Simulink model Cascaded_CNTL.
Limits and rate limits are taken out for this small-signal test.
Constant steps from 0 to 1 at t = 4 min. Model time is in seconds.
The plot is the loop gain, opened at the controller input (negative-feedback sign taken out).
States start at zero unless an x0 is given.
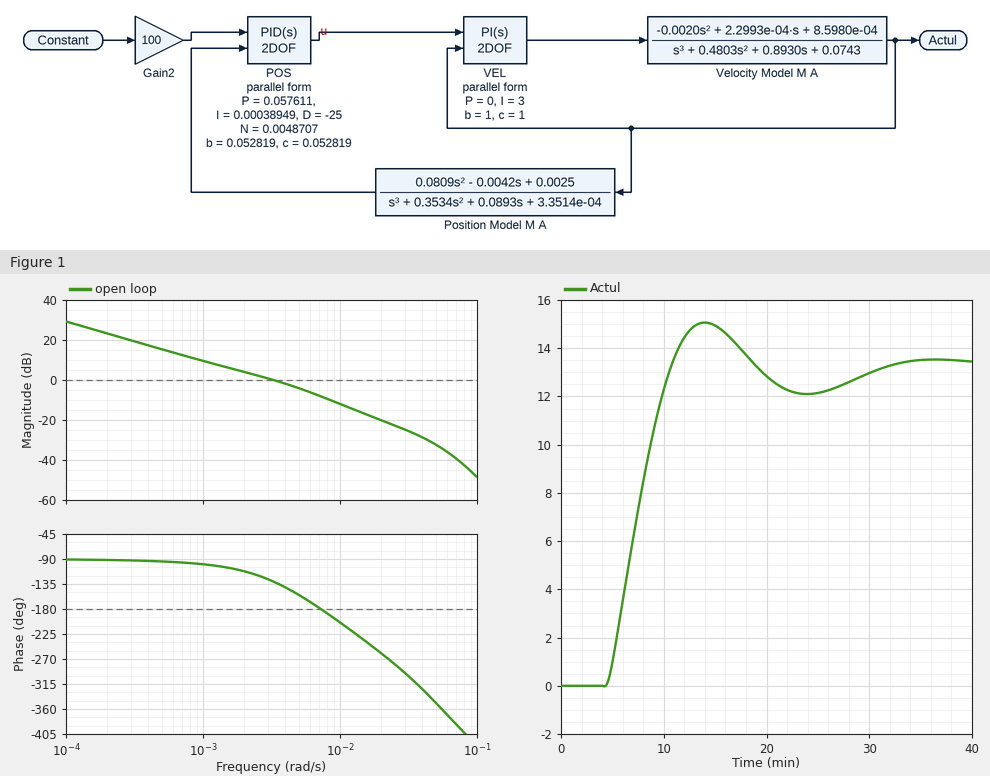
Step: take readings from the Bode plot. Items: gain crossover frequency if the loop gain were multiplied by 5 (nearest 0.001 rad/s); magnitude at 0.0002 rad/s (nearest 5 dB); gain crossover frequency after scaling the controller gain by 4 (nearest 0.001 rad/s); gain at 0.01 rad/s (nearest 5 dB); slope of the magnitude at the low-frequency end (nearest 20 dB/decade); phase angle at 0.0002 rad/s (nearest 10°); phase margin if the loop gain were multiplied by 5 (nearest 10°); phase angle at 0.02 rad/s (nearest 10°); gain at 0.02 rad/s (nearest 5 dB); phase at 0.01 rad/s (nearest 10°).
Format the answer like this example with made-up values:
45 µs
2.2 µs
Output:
0.012 rad/s
25 dB
0.010 rad/s
-10 dB
-20 dB/decade
-90°
-40°
-260°
-20 dB
-200°
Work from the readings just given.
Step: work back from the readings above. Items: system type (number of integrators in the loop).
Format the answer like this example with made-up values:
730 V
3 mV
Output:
1
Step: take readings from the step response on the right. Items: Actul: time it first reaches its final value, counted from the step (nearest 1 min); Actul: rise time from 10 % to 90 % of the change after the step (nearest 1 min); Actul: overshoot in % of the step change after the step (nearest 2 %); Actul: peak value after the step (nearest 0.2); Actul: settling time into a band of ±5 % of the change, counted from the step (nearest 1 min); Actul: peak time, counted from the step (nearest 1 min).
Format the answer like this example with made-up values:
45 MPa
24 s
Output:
7 min
5 min
12 %
15.0
25 min
10 min
